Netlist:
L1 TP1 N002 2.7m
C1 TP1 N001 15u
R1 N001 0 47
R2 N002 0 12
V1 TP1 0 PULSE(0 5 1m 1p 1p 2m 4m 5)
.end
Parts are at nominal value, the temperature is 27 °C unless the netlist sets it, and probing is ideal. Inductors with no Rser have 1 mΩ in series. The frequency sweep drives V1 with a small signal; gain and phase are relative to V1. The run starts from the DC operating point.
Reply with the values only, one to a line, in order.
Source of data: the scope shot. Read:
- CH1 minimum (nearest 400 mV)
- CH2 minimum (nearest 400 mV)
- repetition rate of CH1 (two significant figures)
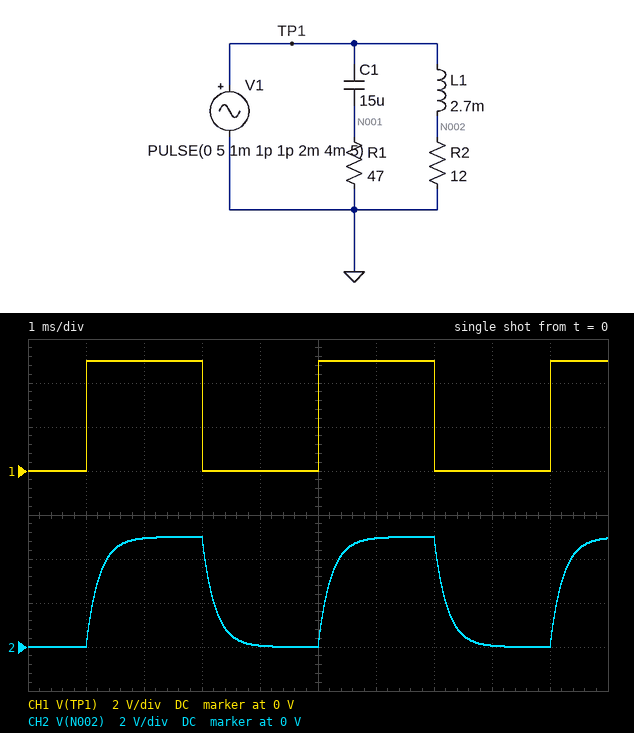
0 V
0 V
250 Hz
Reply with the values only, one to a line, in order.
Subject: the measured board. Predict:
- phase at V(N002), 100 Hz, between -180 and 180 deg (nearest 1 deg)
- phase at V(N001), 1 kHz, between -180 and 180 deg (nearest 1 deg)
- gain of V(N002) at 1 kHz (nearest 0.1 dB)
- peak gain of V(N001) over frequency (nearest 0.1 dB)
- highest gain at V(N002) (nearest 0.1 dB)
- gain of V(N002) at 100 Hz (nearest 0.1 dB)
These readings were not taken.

-8 deg
13 deg
-4.8 dB
0 dB
0 dB
-0.1 dB
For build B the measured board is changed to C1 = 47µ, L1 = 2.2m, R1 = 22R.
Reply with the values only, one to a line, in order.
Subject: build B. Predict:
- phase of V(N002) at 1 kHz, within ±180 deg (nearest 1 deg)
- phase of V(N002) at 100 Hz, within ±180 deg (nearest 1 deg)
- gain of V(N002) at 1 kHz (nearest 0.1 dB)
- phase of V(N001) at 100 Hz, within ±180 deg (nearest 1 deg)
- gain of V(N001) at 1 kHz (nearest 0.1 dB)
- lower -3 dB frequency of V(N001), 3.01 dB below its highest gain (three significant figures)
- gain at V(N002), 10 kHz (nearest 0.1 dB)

-49 deg
-7 deg
-3.7 dB
57 deg
-0.1 dB
154 Hz
-21.3 dB
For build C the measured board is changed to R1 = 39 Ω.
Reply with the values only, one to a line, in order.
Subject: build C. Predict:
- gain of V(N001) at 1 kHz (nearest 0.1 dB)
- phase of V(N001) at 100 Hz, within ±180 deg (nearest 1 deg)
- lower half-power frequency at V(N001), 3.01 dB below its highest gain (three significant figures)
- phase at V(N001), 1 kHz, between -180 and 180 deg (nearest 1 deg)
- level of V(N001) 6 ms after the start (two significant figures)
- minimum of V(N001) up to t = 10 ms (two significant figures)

-0.3 dB
70 deg
272 Hz
15 deg
880 mV
-4.8 V
